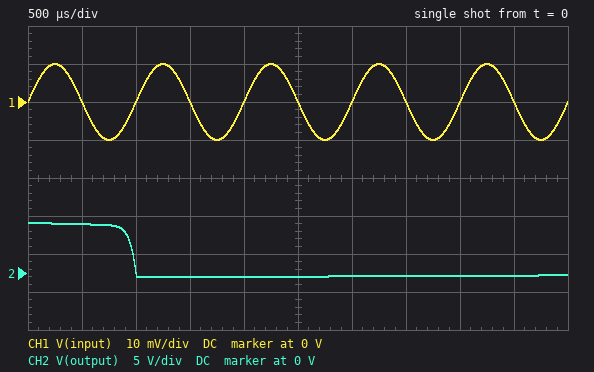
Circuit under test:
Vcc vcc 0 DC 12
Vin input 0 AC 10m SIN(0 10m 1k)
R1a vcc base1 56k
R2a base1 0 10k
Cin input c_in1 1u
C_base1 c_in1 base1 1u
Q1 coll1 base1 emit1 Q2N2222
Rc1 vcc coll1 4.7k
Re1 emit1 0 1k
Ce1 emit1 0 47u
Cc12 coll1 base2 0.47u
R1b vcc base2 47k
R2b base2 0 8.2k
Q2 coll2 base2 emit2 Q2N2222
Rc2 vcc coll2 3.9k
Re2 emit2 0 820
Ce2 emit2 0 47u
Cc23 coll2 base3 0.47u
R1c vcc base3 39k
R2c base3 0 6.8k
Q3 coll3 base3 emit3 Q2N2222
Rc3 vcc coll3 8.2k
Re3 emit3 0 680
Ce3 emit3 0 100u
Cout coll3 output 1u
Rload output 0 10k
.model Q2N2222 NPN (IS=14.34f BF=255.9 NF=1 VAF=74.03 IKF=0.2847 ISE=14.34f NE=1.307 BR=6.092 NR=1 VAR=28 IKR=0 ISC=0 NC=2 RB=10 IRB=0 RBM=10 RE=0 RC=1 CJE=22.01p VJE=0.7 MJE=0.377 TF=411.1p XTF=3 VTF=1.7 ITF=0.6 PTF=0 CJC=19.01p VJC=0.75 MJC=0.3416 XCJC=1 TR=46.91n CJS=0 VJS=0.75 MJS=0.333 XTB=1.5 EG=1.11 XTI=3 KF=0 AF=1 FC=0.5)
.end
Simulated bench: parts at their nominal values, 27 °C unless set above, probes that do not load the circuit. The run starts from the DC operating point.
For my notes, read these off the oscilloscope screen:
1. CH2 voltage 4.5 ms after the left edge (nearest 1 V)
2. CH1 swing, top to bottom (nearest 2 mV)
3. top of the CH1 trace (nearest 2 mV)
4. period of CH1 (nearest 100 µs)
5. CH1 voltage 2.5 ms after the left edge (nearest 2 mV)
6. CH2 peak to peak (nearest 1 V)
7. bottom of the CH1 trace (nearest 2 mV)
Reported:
0 V
20 mV
10 mV
1.0 ms
0 V
7 V
-10 mV
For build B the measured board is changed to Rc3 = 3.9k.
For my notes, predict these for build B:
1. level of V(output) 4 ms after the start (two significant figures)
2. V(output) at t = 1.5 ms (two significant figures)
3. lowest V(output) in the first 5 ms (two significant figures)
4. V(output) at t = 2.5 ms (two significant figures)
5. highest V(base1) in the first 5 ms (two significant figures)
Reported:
-490 mV
-740 mV
-780 mV
-650 mV
890 mV
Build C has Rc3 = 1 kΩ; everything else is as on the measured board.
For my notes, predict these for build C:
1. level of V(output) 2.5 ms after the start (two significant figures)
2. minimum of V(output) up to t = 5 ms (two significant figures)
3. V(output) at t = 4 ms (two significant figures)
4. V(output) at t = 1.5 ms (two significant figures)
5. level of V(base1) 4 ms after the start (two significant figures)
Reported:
-780 mV
-1.0 V
-480 mV
-940 mV
830 mV
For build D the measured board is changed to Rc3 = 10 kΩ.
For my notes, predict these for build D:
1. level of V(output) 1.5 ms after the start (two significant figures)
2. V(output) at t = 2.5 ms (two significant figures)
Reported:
-500 mV
-440 mV
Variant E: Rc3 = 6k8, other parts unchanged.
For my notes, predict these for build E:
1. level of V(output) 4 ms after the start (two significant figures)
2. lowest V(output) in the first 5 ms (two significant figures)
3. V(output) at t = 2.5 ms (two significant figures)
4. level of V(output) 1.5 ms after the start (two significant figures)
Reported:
-410 mV
-630 mV
-530 mV
-600 mV
